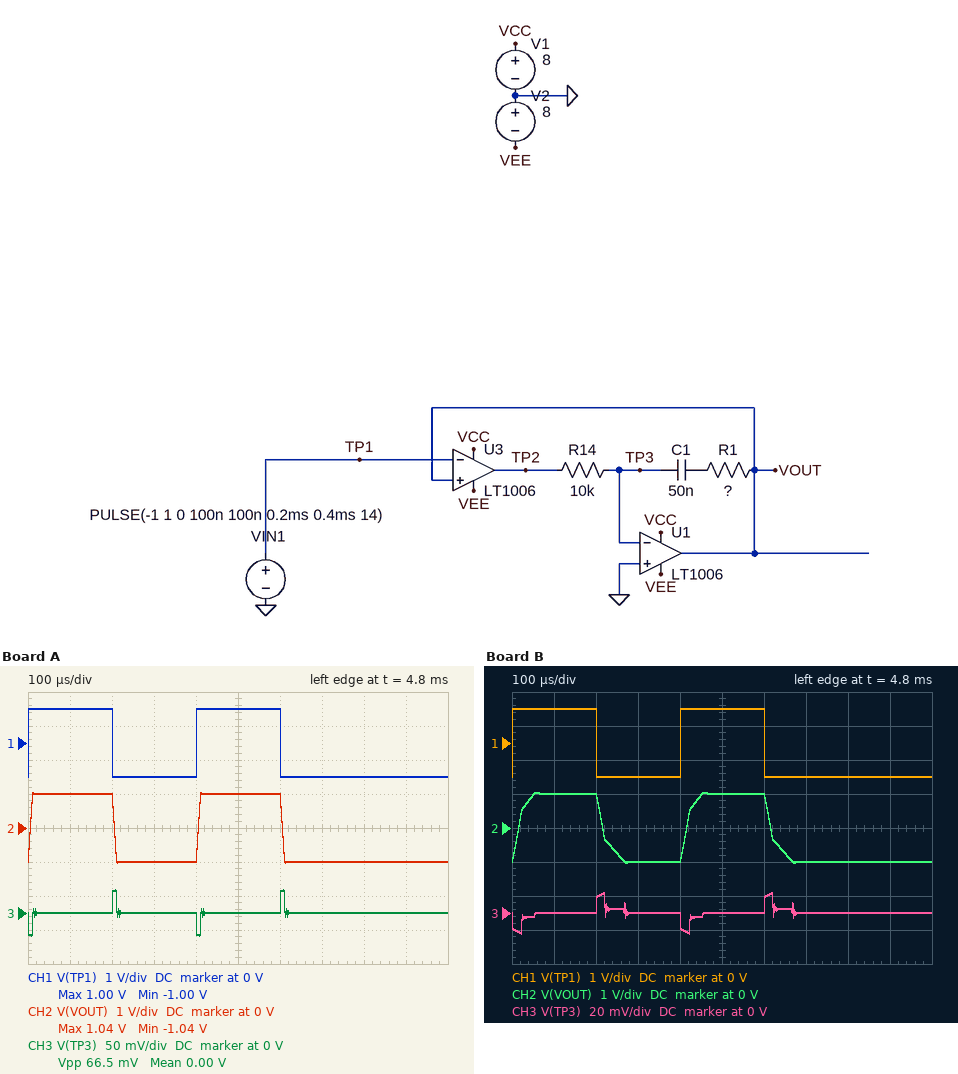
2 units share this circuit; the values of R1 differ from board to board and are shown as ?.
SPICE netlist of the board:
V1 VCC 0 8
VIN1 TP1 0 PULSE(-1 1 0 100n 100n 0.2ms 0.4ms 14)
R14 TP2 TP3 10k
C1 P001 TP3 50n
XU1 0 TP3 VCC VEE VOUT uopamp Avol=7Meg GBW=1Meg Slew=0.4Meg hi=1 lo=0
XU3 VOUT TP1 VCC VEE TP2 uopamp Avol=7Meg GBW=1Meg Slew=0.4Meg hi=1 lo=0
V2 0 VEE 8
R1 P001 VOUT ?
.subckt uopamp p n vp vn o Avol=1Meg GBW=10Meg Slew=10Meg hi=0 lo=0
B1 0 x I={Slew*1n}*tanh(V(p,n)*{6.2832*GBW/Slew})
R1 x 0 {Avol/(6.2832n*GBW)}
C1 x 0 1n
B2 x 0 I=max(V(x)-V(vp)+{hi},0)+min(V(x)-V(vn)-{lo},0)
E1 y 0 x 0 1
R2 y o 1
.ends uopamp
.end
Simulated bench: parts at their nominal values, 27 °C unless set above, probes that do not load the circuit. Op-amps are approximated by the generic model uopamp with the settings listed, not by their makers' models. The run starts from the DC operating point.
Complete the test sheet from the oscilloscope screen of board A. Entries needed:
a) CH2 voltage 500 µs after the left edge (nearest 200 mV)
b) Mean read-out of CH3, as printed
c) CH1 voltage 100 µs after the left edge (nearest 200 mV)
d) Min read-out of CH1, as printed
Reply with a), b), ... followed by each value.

a) 1.0 V
b) 0.00 V
c) 1.0 V
d) -1.00 V
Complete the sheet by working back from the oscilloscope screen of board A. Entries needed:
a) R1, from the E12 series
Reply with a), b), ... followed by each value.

a) 4.7 kΩ
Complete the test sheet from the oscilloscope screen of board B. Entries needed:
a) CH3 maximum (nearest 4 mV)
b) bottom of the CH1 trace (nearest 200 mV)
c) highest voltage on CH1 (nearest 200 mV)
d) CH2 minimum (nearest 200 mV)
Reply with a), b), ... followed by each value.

a) 12 mV
b) -1.0 V
c) 1.0 V
d) -1.0 V
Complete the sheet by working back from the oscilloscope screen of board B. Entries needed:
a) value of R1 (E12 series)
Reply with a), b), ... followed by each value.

a) 1.5 kΩ
